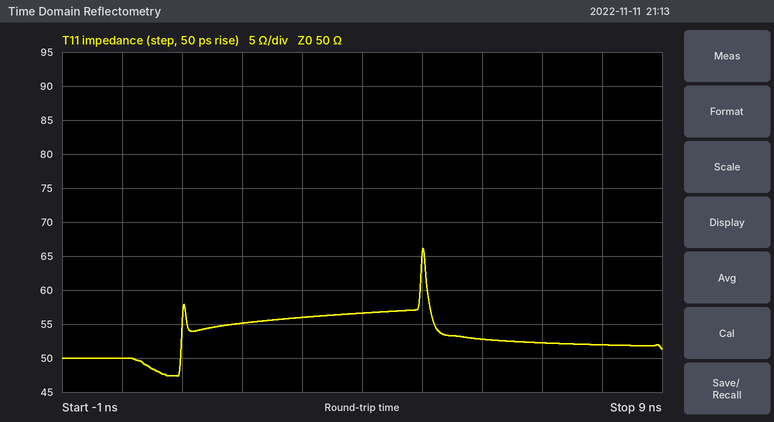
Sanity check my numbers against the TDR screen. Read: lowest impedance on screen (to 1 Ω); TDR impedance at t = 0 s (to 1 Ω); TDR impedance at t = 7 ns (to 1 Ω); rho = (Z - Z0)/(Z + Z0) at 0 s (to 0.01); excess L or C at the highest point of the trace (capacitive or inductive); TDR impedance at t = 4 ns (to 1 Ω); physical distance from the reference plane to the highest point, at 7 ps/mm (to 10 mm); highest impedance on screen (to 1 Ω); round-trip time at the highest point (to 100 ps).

47 Ω
50 Ω
52 Ω
0.00
inductive
57 Ω
360 mm
66 Ω
5.0 ns
